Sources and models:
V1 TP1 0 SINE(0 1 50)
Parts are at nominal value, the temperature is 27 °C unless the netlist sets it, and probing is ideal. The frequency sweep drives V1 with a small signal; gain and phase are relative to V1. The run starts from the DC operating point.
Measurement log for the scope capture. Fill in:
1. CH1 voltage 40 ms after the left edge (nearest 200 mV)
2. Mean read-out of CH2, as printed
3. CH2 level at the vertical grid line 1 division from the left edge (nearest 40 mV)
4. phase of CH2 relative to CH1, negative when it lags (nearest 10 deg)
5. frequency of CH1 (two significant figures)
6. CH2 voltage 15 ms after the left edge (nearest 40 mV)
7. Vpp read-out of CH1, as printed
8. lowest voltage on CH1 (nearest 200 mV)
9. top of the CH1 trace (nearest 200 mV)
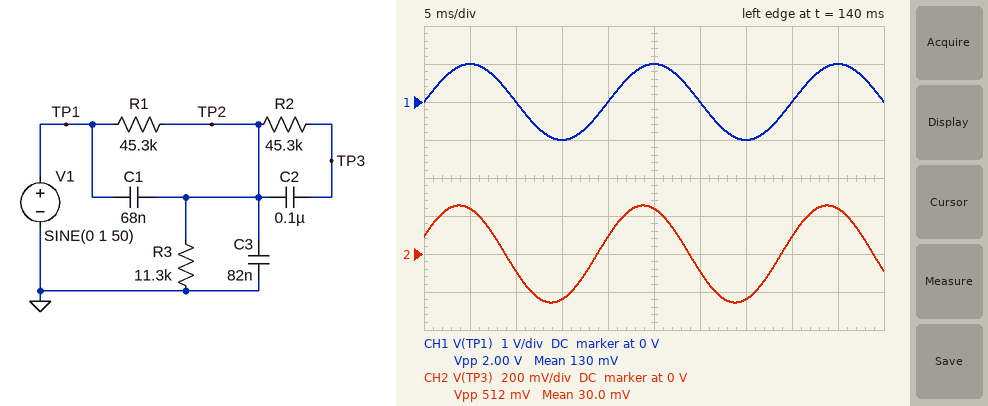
0 V
30.0 mV
240 mV
20 deg
50 Hz
-240 mV
2.00 V
-1.0 V
1.0 V
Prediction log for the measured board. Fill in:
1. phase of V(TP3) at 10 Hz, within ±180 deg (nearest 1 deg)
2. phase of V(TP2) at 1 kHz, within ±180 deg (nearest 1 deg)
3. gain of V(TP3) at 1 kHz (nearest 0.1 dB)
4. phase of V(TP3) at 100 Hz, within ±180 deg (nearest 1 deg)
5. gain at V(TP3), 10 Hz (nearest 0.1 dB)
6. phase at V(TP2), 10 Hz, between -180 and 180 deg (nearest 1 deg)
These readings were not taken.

6 deg
4 deg
-6.9 dB
22 deg
-13.9 dB
6 deg
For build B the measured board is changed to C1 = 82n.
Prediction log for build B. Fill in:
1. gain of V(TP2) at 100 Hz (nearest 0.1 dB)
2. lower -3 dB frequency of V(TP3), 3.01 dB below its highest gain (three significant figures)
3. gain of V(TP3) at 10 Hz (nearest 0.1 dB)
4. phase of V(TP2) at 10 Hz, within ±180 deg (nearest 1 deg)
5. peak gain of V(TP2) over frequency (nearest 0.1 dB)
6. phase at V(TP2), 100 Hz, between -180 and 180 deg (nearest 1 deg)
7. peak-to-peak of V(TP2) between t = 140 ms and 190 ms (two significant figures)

-8.6 dB
88.6 Hz
-13.8 dB
8 deg
-6.0 dB
24 deg
560 mV
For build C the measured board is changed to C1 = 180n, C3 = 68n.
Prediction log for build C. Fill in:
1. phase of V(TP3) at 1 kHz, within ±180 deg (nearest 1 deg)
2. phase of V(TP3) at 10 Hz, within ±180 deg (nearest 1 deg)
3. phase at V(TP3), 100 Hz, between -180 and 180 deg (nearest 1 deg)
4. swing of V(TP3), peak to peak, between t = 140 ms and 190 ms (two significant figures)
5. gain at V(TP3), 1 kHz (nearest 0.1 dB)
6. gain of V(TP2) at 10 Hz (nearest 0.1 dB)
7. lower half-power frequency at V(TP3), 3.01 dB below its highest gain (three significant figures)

3 deg
19 deg
24 deg
900 mV
-2.8 dB
-13.1 dB
65.4 Hz
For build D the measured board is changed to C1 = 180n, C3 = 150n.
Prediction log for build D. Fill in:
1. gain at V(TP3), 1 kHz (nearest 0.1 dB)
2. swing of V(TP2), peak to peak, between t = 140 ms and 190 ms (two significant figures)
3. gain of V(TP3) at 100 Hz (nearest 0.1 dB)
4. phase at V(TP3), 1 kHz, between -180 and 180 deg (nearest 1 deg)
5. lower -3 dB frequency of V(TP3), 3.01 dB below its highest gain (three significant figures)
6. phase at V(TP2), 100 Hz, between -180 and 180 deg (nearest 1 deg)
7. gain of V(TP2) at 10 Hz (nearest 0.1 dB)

-5.3 dB
800 mV
-6.2 dB
2 deg
45.6 Hz
17 deg
-13.1 dB
